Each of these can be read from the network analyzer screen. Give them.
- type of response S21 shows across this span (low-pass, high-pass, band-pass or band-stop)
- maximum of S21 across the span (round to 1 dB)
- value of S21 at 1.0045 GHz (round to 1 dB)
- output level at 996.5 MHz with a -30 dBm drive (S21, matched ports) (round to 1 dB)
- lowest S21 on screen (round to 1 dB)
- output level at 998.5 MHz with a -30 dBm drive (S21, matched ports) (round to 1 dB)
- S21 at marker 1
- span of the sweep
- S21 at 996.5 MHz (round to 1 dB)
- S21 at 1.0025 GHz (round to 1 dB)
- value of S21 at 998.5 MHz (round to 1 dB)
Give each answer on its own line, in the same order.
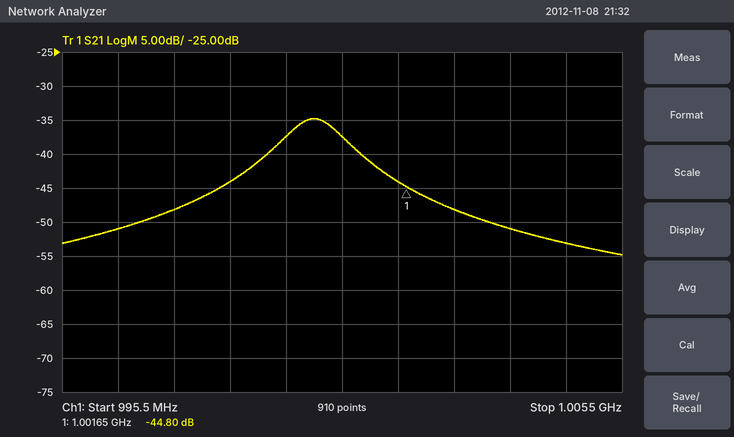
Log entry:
band-pass
-35 dB
-53 dB
-81 dBm
-55 dB
-74 dBm
-44.80 dB
10 MHz
-51 dB
-48 dB
-44 dB
